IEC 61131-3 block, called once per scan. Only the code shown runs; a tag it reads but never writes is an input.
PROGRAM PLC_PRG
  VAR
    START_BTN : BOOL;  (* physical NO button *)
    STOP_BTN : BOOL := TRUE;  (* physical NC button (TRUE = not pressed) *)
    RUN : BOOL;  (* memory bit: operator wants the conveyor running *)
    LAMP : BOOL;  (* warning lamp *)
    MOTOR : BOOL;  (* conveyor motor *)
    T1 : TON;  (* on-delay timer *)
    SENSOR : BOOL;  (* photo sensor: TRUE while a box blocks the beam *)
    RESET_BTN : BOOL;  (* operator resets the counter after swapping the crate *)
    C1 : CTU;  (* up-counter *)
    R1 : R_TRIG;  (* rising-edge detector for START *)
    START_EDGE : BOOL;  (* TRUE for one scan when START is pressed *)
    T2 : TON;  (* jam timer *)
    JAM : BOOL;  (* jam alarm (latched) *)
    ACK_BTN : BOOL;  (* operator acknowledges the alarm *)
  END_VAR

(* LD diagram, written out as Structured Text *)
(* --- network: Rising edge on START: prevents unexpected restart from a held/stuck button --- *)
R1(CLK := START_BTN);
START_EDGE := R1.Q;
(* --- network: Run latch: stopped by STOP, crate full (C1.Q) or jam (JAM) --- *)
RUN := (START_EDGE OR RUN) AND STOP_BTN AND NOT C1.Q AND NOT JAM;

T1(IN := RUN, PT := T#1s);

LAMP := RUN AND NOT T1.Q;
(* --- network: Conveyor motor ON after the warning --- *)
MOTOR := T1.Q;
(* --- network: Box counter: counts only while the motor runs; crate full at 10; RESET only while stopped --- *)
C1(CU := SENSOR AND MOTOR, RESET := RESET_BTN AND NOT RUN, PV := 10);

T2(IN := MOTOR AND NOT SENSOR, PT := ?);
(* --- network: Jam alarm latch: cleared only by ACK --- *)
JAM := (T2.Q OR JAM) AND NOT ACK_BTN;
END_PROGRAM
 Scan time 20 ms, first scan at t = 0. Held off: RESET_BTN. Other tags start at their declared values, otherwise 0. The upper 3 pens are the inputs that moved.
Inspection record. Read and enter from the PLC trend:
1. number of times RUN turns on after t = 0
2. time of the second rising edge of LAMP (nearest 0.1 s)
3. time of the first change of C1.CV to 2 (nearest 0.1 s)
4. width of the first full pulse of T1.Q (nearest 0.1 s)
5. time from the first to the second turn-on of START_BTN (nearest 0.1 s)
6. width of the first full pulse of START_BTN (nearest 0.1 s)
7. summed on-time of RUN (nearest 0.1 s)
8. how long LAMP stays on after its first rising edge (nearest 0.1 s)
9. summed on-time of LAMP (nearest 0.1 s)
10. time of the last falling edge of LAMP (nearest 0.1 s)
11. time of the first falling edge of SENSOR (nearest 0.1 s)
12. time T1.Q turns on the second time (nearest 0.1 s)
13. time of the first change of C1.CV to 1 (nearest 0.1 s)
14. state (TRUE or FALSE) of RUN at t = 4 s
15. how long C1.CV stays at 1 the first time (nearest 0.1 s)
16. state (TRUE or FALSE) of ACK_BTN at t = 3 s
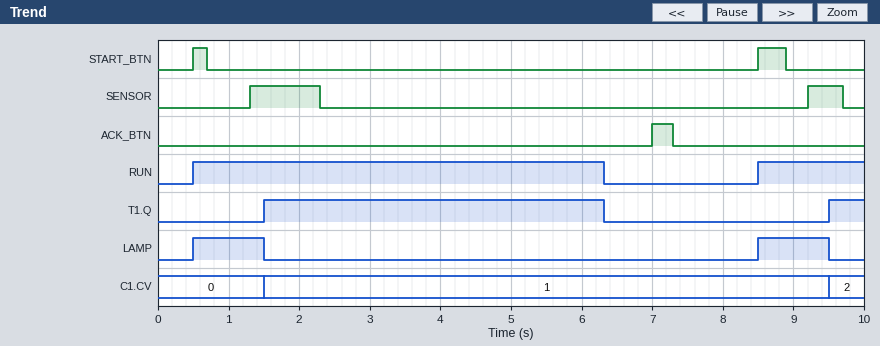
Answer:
2
8.5 s
9.5 s
4.8 s
8.0 s
0.2 s
7.3 s
1.0 s
2.0 s
9.5 s
2.3 s
9.5 s
1.5 s
TRUE
8.0 s
FALSE
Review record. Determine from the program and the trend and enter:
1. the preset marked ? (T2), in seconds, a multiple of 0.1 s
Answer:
4.0 s
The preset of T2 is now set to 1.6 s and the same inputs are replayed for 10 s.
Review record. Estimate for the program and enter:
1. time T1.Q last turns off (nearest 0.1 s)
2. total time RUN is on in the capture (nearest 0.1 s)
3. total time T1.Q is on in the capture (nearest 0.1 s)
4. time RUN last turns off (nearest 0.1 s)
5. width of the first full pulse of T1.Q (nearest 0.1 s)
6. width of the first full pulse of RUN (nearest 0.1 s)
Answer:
3.9 s
4.9 s
2.9 s
3.9 s
2.4 s
3.4 s
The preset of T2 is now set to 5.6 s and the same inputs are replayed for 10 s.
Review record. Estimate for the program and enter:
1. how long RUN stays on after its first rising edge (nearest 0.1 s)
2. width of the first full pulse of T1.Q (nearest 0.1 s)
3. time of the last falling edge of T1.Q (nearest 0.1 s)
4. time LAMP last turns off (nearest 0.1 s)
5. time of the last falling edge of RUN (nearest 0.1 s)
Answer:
7.4 s
6.4 s
7.9 s
1.5 s
7.9 s
